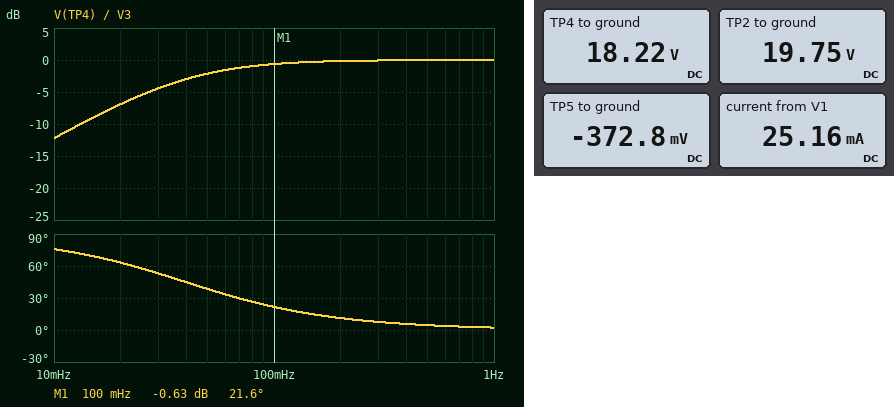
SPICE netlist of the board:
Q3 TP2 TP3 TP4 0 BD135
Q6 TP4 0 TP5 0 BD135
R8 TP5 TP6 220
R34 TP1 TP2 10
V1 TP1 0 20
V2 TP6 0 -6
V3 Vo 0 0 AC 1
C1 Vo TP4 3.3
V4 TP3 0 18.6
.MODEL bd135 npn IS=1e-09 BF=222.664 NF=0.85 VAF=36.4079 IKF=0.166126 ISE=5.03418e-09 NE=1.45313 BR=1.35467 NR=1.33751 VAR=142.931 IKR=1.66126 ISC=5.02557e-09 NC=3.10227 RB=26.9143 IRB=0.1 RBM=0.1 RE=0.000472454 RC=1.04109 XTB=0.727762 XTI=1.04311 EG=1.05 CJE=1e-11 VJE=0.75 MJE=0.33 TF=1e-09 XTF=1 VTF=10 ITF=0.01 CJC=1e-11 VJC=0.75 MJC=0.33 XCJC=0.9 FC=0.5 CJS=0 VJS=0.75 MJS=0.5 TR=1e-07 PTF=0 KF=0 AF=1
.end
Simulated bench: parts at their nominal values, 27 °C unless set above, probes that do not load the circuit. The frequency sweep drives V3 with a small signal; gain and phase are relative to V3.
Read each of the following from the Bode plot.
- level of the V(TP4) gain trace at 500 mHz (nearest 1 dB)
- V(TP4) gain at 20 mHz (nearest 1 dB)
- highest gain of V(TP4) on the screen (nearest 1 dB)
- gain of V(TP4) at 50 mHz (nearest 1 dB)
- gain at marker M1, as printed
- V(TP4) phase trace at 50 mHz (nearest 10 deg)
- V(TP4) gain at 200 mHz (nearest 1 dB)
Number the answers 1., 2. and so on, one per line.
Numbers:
1. 0 dB
2. -7 dB
3. 0 dB
4. -2 dB
5. -0.63 dB
6. 40 deg
7. 0 dB
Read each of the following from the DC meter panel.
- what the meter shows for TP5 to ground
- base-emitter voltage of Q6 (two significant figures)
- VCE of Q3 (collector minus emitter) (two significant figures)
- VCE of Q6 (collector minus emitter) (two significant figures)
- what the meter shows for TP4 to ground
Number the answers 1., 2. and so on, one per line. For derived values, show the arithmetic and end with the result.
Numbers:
1. -372.8 mV
2. 0 V - (-372.8 mV) = 370 mV
3. 19.75 V - 18.22 V = 1.5 V
4. 18.22 V - (-372.8 mV) = 19 V
5. 18.22 V
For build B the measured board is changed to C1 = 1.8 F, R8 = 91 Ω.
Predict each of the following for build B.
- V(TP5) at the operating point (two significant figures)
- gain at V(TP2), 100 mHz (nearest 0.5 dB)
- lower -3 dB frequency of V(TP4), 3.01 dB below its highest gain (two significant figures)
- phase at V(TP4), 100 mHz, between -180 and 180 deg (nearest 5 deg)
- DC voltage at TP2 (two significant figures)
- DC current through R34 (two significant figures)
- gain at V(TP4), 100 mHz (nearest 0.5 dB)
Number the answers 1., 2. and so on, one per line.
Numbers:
1. -400 mV
2. 18.5 dB
3. 120 mHz
4. 50 deg
5. 19 V
6. 61 mA
7. -4.0 dB
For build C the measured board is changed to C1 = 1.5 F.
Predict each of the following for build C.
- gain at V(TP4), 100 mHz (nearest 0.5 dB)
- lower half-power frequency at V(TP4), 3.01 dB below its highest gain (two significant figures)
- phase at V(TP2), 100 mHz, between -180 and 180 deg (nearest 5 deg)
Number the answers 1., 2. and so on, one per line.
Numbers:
1. -2.5 dB
2. 87 mHz
3. 40 deg
